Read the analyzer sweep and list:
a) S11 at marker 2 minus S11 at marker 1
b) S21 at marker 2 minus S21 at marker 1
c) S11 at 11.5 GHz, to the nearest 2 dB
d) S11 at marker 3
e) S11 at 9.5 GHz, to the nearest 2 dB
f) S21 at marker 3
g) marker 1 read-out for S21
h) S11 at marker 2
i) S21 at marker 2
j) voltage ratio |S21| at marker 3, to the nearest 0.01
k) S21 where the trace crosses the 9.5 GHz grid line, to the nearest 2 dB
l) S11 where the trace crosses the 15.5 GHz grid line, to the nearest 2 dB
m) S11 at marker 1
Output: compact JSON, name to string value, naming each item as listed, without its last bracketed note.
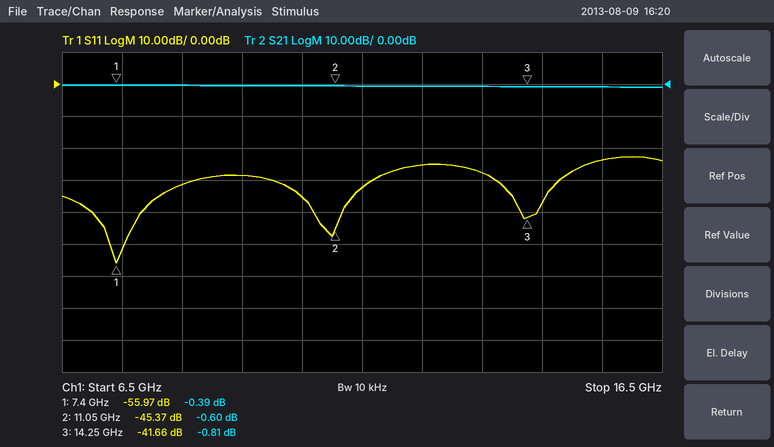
{"S11 at marker 2 minus S11 at marker 1": "10.60 dB", "S21 at marker 2 minus S21 at marker 1": "-0.21 dB", "S11 at 11.5 GHz, to the nearest 2 dB": "-32 dB", "S11 at marker 3": "-41.66 dB", "S11 at 9.5 GHz, to the nearest 2 dB": "-28 dB", "S21 at marker 3": "-0.81 dB", "marker 1 read-out for S21": "-0.39 dB", "S11 at marker 2": "-45.37 dB", "S21 at marker 2": "-0.60 dB", "voltage ratio |S21| at marker 3, to the nearest 0.01": "0.91", "S21 where the trace crosses the 9.5 GHz grid line, to the nearest 2 dB": "0 dB", "S11 where the trace crosses the 15.5 GHz grid line, to the nearest 2 dB": "-24 dB", "S11 at marker 1": "-55.97 dB"}
